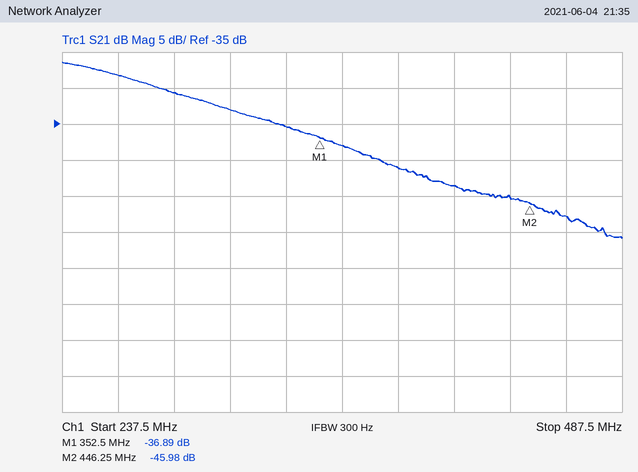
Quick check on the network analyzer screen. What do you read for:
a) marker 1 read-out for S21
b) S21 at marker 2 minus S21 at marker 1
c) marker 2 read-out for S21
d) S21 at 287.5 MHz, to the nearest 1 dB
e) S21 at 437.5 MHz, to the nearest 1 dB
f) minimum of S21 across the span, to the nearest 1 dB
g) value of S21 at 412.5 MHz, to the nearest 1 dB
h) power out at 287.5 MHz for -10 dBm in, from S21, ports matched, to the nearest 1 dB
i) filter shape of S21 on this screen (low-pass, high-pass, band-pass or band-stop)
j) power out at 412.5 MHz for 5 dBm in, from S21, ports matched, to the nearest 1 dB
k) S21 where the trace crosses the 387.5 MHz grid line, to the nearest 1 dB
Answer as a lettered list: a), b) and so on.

a) -36.89 dB
b) -9.09 dB
c) -45.98 dB
d) -31 dB
e) -45 dB
f) -51 dB
g) -44 dB
h) -41 dBm
i) low-pass
j) -39 dBm
k) -41 dB
